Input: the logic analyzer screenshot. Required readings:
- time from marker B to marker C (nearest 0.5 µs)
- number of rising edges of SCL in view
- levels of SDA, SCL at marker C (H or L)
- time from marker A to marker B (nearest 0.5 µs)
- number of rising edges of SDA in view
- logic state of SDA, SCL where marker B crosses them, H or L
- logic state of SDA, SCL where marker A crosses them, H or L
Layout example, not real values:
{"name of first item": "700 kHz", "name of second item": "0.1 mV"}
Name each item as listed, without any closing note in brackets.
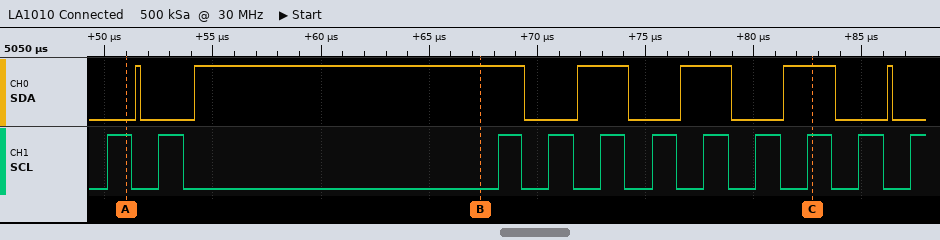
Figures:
{"time from marker B to marker C": "15.5 µs", "number of rising edges of SCL in view": "11", "levels of SDA, SCL at marker C": "SDA=H, SCL=H", "time from marker A to marker B": "16.5 µs", "number of rising edges of SDA in view": "6", "logic state of SDA, SCL where marker B crosses them, H or L": "SDA=H, SCL=L", "logic state of SDA, SCL where marker A crosses them, H or L": "SDA=L, SCL=H"}
